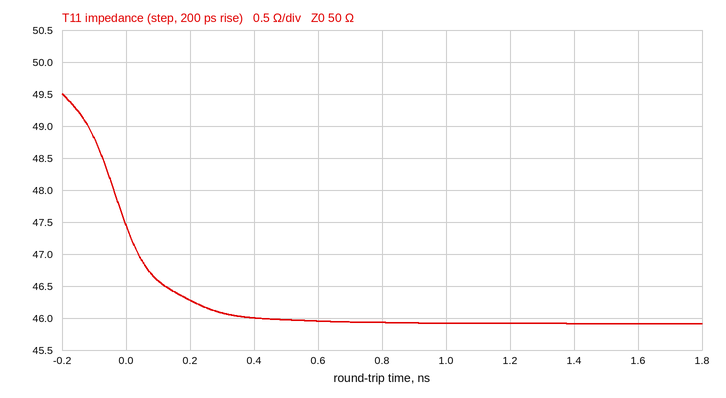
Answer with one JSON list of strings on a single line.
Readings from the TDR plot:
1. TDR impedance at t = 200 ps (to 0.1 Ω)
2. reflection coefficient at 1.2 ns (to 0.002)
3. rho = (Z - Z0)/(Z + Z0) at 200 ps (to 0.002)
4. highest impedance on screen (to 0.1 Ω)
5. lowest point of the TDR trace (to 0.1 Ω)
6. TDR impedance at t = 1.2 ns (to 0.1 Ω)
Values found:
["46.3 Ω", "-0.042", "-0.038", "49.5 Ω", "45.9 Ω", "45.9 Ω"]
